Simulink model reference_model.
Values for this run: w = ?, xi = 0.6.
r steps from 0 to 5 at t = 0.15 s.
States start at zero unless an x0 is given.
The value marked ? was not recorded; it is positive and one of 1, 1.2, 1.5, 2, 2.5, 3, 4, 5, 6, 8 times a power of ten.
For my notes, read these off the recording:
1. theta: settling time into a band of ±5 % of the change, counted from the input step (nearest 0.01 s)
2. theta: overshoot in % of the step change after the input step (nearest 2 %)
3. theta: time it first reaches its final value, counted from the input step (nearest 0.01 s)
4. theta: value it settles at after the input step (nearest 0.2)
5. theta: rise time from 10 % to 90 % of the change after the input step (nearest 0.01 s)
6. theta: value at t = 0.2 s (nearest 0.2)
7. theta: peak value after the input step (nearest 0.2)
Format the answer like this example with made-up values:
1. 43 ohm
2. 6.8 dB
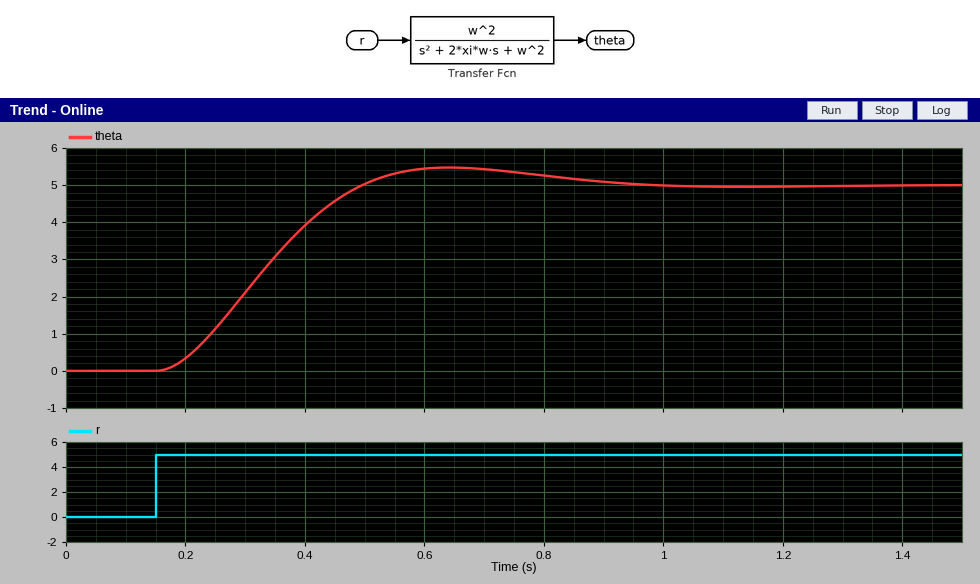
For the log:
1. 0.65 s
2. 10 %
3. 0.35 s
4. 5.0
5. 0.23 s
6. 0.4
7. 5.4
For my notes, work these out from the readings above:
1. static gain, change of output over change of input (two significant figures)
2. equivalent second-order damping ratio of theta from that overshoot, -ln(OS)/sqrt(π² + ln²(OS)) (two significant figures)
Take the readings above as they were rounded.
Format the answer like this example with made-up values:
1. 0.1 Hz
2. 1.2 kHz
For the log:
1. 1.0
2. 0.59
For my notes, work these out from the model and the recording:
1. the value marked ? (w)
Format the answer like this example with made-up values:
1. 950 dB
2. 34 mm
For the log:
1. 8
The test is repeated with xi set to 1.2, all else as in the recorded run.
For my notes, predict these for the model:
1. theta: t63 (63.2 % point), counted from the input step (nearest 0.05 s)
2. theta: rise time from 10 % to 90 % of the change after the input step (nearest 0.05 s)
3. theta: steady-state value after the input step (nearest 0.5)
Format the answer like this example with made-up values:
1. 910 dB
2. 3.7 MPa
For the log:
1. 0.30 s
2. 0.55 s
3. 5.0
